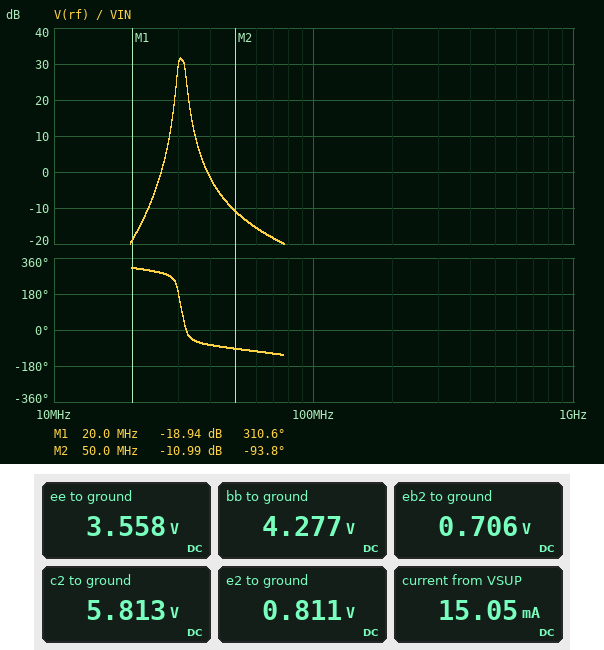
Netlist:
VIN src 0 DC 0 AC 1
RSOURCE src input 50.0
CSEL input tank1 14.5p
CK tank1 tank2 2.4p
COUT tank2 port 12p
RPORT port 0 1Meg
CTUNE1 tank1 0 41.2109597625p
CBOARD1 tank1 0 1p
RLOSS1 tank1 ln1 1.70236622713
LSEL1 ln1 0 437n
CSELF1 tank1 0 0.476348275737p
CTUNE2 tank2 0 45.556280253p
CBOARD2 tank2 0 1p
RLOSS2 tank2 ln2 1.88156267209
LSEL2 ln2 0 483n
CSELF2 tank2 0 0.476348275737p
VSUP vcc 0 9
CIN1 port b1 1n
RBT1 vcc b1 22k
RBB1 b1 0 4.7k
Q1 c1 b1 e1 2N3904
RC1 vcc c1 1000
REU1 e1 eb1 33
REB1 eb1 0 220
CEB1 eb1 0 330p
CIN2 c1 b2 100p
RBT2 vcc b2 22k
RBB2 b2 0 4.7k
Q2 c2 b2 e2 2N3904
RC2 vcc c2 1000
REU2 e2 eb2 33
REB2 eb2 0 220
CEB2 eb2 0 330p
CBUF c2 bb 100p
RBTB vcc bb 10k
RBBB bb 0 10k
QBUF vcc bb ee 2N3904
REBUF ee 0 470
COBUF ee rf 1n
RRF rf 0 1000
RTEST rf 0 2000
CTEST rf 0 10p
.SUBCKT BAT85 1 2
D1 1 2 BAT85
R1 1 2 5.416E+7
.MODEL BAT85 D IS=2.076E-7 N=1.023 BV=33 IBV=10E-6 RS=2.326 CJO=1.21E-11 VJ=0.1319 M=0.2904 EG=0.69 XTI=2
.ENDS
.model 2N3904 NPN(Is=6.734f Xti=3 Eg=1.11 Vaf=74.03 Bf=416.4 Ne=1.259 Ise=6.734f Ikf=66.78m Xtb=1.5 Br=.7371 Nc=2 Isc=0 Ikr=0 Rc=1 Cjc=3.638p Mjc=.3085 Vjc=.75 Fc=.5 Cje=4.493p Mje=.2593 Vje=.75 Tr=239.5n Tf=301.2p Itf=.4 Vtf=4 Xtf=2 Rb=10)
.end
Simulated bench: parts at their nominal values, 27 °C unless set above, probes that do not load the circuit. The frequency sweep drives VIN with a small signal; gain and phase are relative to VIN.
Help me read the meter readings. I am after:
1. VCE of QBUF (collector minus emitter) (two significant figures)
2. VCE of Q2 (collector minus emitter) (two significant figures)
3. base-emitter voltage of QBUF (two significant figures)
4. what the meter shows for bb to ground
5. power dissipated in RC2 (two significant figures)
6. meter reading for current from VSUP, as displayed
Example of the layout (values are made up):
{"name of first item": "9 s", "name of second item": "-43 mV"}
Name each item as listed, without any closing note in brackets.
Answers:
{"VCE of QBUF (collector minus emitter)": "5.4 V", "VCE of Q2 (collector minus emitter)": "5.0 V", "base-emitter voltage of QBUF": "720 mV", "what the meter shows for bb to ground": "4.277 V", "power dissipated in RC2": "10 mW", "meter reading for current from VSUP, as displayed": "15.05 mA"}
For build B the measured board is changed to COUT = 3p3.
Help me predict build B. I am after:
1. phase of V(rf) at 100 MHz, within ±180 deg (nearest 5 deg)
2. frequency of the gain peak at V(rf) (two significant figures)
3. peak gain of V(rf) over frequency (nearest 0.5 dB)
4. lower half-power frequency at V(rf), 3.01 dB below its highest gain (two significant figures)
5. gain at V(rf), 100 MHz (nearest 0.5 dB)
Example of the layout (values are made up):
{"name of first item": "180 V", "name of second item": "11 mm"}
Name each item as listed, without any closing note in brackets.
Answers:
{"phase of V(rf) at 100 MHz, within ±180 deg": "-140 deg", "frequency of the gain peak at V(rf)": "32 MHz", "peak gain of V(rf) over frequency": "27.0 dB", "lower half-power frequency at V(rf), 3.01 dB below its highest gain": "31 MHz", "gain at V(rf), 100 MHz": "-31.0 dB"}
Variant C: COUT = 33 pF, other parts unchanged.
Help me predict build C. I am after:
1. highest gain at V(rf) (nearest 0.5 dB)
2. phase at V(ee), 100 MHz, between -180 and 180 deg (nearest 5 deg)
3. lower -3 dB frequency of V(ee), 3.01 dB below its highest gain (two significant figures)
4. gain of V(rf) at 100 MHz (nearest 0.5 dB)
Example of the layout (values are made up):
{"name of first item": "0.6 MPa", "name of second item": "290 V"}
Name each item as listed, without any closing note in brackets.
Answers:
{"highest gain at V(rf)": "30.0 dB", "phase at V(ee), 100 MHz, between -180 and 180 deg": "-150 deg", "lower -3 dB frequency of V(ee), 3.01 dB below its highest gain": "29 MHz", "gain of V(rf) at 100 MHz": "-21.0 dB"}
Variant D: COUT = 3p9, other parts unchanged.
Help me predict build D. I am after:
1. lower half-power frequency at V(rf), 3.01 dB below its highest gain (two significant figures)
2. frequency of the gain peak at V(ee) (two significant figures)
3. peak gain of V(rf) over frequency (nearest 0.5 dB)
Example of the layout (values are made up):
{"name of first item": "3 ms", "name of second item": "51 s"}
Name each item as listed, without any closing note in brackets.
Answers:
{"lower half-power frequency at V(rf), 3.01 dB below its highest gain": "31 MHz", "frequency of the gain peak at V(ee)": "32 MHz", "peak gain of V(rf) over frequency": "28.0 dB"}
